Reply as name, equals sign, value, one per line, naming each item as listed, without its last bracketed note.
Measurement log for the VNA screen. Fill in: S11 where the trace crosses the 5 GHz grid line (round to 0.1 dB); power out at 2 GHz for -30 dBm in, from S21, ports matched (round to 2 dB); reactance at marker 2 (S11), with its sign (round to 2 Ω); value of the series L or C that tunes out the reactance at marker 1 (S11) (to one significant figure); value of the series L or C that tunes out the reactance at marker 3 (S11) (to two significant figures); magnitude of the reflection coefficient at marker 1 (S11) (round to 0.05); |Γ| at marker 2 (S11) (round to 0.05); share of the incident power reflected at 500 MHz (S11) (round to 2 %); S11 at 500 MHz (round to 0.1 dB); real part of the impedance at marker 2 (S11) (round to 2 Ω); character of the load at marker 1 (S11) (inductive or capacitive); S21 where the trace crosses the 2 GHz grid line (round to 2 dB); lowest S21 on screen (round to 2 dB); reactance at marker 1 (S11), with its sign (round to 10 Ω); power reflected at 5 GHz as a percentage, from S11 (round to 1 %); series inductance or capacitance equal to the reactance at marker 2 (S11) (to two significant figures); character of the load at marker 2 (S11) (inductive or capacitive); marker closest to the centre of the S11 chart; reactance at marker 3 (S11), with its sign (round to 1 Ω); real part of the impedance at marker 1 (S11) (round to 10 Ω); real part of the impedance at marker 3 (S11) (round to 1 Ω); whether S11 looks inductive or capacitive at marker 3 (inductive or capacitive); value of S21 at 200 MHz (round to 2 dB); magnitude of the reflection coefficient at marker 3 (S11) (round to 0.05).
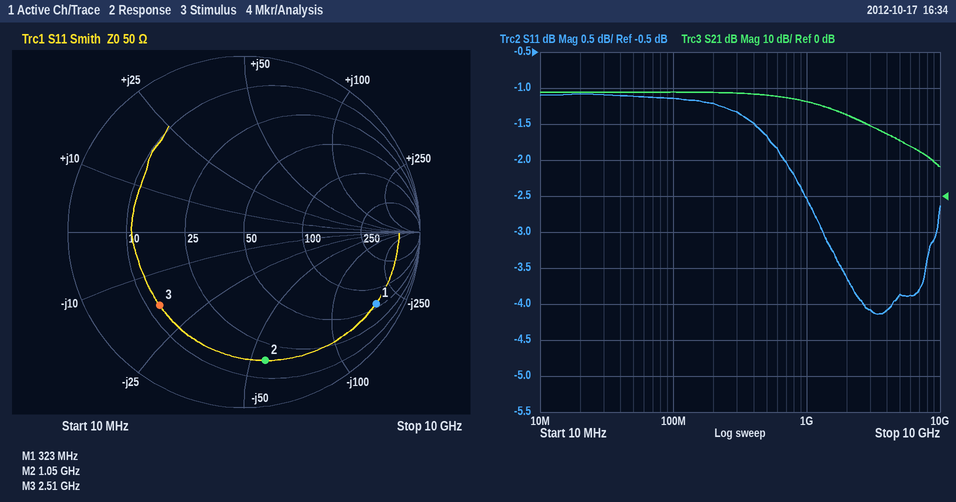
S11 where the trace crosses the 5 GHz grid line = -3.9 dB
power out at 2 GHz for -30 dBm in, from S21, ports matched = -8 dBm
reactance at marker 2 (S11), with its sign = -56 Ω
value of the series L or C that tunes out the reactance at marker 1 (S11) = 90 nH
value of the series L or C that tunes out the reactance at marker 3 (S11) = 1.1 nH
magnitude of the reflection coefficient at marker 1 (S11) = 0.85
|Γ| at marker 2 (S11) = 0.75
share of the incident power reflected at 500 MHz (S11) = 68 %
S11 at 500 MHz = -1.7 dB
real part of the impedance at marker 2 (S11) = 18 Ω
character of the load at marker 1 (S11) = capacitive
S21 where the trace crosses the 2 GHz grid line = 22 dB
lowest S21 on screen = 8 dB
reactance at marker 1 (S11), with its sign = -180 Ω
power reflected at 5 GHz as a percentage, from S11 = 41 %
series inductance or capacitance equal to the reactance at marker 2 (S11) = 2.7 pF
character of the load at marker 2 (S11) = capacitive
marker closest to the centre of the S11 chart = marker 3
reactance at marker 3 (S11), with its sign = -18 Ω
real part of the impedance at marker 1 (S11) = 60 Ω
real part of the impedance at marker 3 (S11) = 13 Ω
whether S11 looks inductive or capacitive at marker 3 = capacitive
value of S21 at 200 MHz = 28 dB
magnitude of the reflection coefficient at marker 3 (S11) = 0.65
